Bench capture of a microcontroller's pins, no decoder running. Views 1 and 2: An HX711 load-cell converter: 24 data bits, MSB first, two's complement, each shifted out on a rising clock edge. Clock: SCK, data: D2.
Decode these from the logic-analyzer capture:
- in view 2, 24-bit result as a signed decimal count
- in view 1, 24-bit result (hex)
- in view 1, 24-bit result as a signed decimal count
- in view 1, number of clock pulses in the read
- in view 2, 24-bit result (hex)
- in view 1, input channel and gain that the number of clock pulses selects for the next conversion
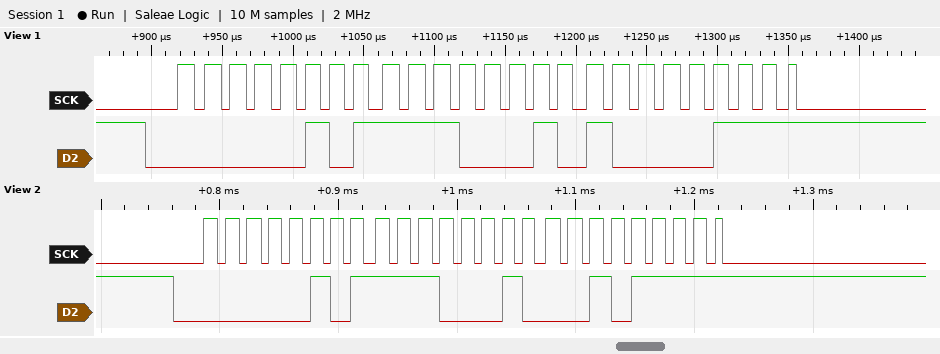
385583
0x05E287
385671
25
0x05E22F
channel A, gain 128
